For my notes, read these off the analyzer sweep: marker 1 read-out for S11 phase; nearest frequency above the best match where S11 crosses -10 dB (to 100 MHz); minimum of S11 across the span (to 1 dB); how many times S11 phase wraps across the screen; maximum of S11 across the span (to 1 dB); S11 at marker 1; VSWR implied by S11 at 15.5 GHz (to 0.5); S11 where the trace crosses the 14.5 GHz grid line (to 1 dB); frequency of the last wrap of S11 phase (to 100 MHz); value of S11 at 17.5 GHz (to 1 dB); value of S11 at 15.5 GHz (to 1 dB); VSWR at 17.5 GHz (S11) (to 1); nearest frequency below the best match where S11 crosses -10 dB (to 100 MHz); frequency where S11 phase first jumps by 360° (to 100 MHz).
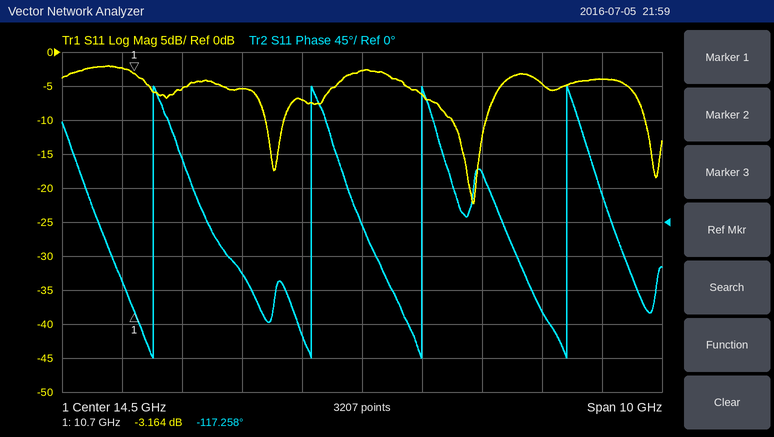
-117.258°
16.6 GHz
-22 dB
4
-2 dB
-3.164 dB
3.0
-3 dB
17.9 GHz
-5 dB
-6 dB
4
16.0 GHz
11.0 GHz
